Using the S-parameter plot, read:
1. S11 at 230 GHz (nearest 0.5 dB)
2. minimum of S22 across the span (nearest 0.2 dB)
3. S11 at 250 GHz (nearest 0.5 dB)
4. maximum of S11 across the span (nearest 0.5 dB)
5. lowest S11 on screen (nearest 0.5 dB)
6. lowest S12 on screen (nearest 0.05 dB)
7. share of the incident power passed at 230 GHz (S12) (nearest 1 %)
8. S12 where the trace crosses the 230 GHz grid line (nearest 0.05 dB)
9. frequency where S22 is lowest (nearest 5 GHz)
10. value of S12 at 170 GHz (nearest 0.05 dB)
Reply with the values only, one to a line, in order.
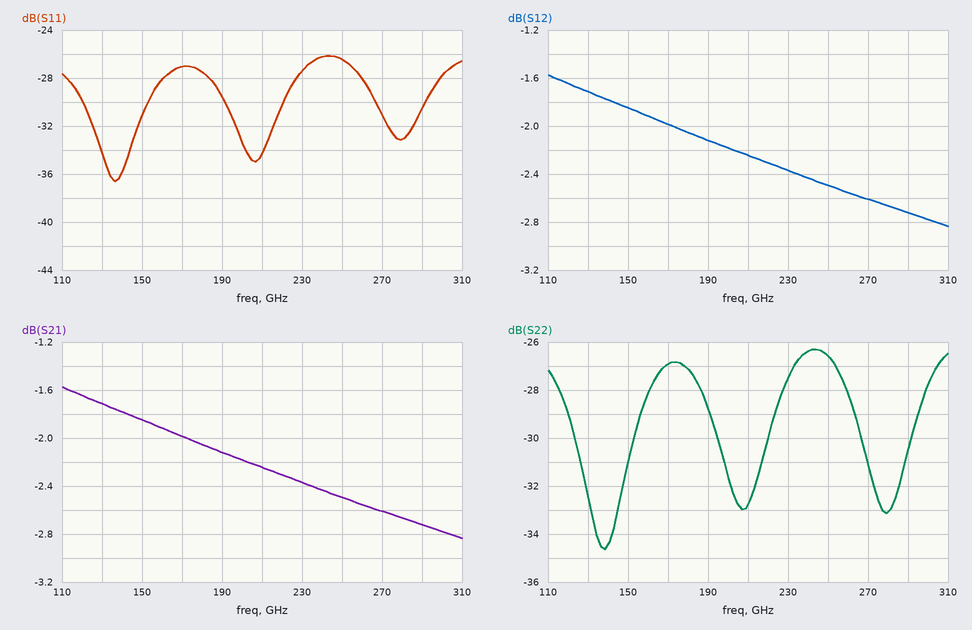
-27.5 dB
-34.6 dB
-26.5 dB
-26.0 dB
-36.5 dB
-2.85 dB
58 %
-2.35 dB
140 GHz
-2.00 dB
